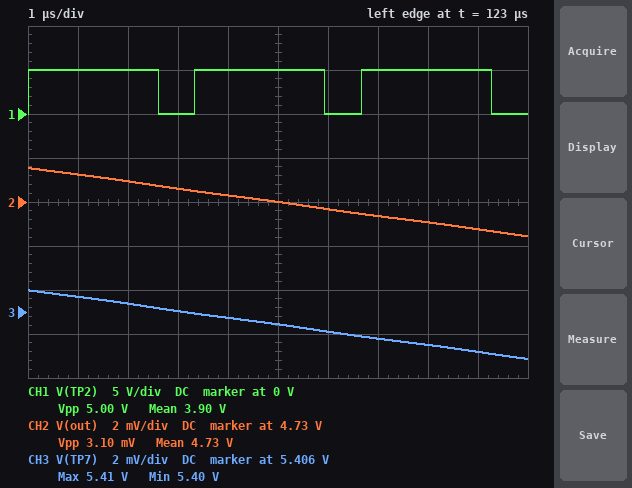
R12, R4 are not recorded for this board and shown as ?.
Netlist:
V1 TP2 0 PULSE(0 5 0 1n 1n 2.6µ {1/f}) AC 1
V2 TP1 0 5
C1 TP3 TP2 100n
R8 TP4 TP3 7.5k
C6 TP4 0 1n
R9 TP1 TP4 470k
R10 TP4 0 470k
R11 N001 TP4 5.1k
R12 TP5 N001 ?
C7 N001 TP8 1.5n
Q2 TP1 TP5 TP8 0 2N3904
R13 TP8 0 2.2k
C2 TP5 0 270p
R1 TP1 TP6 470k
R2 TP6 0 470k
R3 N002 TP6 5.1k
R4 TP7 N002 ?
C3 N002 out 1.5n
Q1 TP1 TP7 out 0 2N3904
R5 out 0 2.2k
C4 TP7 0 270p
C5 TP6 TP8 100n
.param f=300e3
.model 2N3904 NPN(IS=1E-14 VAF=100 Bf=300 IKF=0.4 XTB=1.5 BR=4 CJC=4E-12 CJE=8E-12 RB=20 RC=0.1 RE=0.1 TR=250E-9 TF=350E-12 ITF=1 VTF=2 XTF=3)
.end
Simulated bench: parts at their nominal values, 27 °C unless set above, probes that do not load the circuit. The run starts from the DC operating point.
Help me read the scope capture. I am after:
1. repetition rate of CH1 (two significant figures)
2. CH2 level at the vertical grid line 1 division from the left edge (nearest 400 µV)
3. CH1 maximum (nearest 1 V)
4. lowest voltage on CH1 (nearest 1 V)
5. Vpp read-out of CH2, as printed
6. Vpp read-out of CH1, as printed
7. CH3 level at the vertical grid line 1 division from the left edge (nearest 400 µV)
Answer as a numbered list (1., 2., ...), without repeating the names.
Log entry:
1. 300 kHz
2. 4.7312 V
3. 5 V
4. 0 V
5. 3.10 mV
6. 5.00 V
7. 5.4068 V
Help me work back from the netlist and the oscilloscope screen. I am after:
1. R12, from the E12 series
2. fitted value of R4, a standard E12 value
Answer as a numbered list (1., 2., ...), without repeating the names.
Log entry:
1. 22 kΩ
2. 3.9 kΩ
